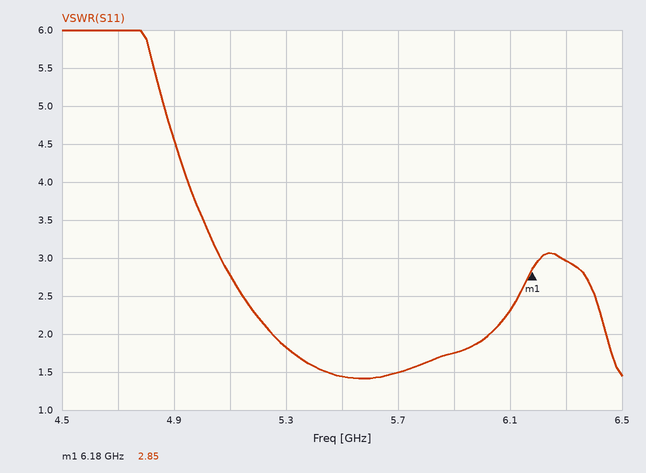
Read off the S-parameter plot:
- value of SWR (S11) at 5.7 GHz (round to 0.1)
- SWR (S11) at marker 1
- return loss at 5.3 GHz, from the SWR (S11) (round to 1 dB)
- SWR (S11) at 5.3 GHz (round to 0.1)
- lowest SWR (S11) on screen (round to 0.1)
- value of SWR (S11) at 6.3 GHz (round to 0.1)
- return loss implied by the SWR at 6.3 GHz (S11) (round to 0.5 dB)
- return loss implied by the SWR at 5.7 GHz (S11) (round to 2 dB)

1.5
2.85
11 dB
1.8
1.4
3.0
6.0 dB
14 dB
